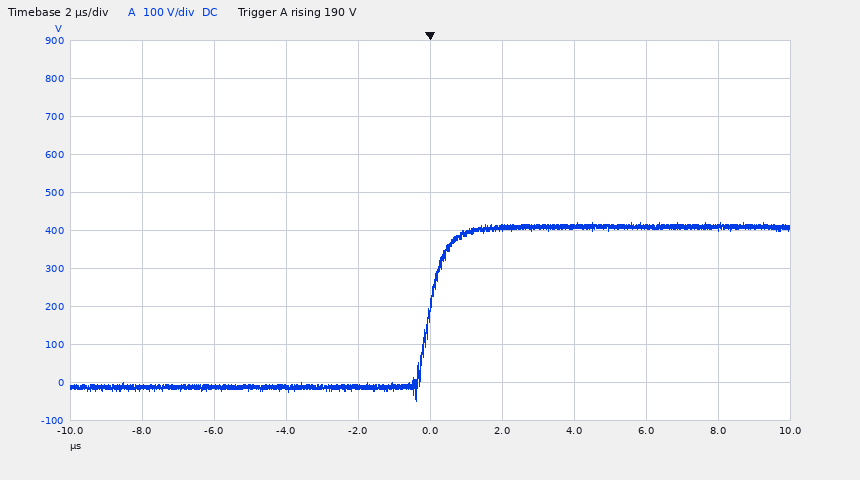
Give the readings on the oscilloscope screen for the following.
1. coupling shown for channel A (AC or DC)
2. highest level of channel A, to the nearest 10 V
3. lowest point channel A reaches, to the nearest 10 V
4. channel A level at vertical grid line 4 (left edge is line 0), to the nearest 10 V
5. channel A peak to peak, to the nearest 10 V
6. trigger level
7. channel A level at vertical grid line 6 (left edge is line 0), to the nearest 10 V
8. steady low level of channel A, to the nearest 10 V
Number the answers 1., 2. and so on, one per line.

1. DC
2. 420 V
3. -50 V
4. -10 V
5. 470 V
6. 190 V
7. 410 V
8. -10 V
